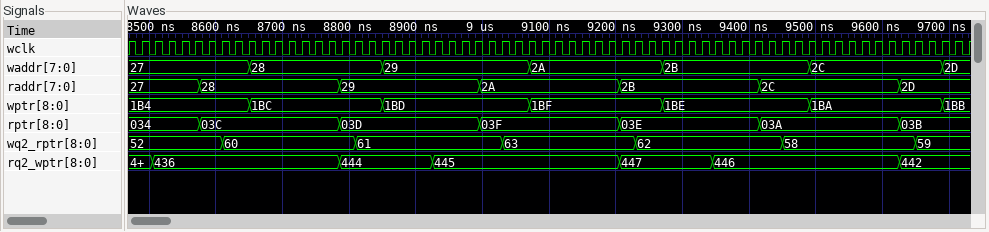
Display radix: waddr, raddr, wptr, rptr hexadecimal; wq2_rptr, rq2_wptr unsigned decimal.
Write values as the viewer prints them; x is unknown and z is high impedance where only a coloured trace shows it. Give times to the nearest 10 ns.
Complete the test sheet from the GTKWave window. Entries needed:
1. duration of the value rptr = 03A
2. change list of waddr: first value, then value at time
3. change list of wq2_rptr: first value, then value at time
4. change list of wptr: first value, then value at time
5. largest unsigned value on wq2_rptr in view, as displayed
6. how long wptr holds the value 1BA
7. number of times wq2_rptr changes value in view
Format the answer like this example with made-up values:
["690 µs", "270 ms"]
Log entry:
["210 ns", "27, 28 at 8650 ns, 29 at 8850 ns, 2A at 9070 ns, 2B at 9270 ns, 2C at 9490 ns, 2D at 9690 ns", "52, 60 at 8610 ns, 61 at 8810 ns, 63 at 9030 ns, 62 at 9230 ns, 58 at 9450 ns, 59 at 9650 ns", "1B4, 1BC at 8650 ns, 1BD at 8850 ns, 1BF at 9070 ns, 1BE at 9270 ns, 1BA at 9490 ns, 1BB at 9690 ns", "63", "200 ns", "6"]
